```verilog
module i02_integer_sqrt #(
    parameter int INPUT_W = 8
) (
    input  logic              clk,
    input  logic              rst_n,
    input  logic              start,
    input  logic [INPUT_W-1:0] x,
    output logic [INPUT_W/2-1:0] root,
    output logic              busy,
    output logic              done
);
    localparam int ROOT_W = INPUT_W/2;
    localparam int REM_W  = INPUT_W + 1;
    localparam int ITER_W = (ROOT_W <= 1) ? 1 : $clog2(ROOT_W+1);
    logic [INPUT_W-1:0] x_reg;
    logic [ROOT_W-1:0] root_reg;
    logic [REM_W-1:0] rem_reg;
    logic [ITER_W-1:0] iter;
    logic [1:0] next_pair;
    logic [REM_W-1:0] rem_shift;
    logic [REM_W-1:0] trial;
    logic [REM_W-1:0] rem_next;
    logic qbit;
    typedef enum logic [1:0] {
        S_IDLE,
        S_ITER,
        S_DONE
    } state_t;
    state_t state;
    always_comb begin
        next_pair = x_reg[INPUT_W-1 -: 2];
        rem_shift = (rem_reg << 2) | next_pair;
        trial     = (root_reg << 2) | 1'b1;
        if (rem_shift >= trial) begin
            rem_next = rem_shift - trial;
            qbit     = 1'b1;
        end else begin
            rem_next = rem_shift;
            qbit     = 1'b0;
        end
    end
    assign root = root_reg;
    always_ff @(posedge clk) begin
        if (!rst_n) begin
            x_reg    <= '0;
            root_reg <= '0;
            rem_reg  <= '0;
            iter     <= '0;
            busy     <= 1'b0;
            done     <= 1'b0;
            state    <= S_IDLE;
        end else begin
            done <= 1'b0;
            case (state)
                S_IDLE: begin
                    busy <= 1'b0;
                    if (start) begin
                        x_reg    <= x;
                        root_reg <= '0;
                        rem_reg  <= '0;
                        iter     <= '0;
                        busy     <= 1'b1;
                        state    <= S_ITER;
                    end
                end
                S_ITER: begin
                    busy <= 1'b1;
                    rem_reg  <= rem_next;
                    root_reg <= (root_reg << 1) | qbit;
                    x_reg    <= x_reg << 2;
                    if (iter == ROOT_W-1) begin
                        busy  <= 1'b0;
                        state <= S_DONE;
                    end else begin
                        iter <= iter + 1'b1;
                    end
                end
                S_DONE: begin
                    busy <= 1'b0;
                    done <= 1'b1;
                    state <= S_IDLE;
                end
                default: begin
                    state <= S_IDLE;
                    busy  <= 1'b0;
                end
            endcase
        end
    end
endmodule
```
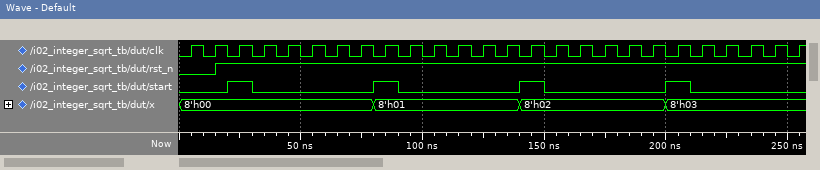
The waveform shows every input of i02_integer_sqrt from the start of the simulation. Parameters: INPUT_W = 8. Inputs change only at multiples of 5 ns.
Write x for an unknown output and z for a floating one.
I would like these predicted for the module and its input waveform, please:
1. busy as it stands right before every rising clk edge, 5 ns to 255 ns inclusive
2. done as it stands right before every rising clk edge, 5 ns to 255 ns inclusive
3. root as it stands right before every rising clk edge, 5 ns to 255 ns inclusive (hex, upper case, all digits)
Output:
x 0 0 1 1 1 1 0 0 1 1 1 1 0 0 1 1 1 1 0 0 1 1 1 1 0
x 0 0 0 0 0 0 0 1 0 0 0 0 0 1 0 0 0 0 0 1 0 0 0 0 0
x, 0, 0, 0, 0, 0, 0, 0, 0, 0, 0, 0, 0, 1, 1, 0, 0, 0, 0, 1, 1, 0, 0, 0, 0, 1
